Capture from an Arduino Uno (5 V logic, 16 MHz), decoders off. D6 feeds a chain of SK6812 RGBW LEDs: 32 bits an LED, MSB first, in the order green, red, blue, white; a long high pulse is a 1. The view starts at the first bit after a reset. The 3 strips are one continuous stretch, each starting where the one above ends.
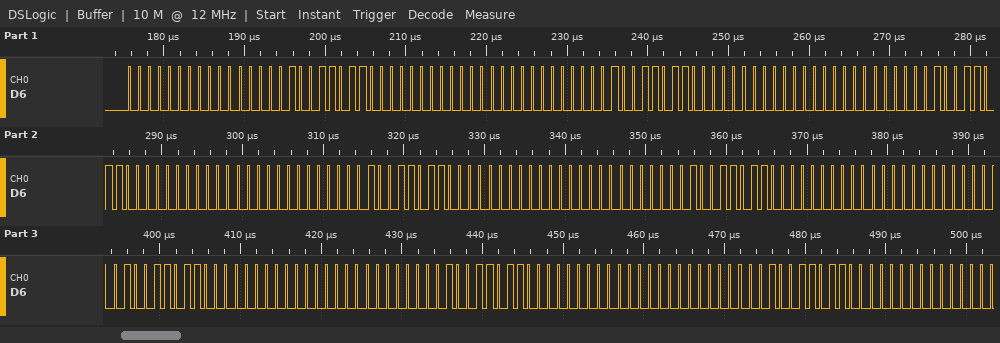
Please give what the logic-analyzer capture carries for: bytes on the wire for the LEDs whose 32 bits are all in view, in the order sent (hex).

00 00 9B 00 00 00 9B 00 00 00 9B 00 00 00 9B 00 00 00 9B 00 00 00 9B 00 00 00 9B 00 00 00 9B 00
